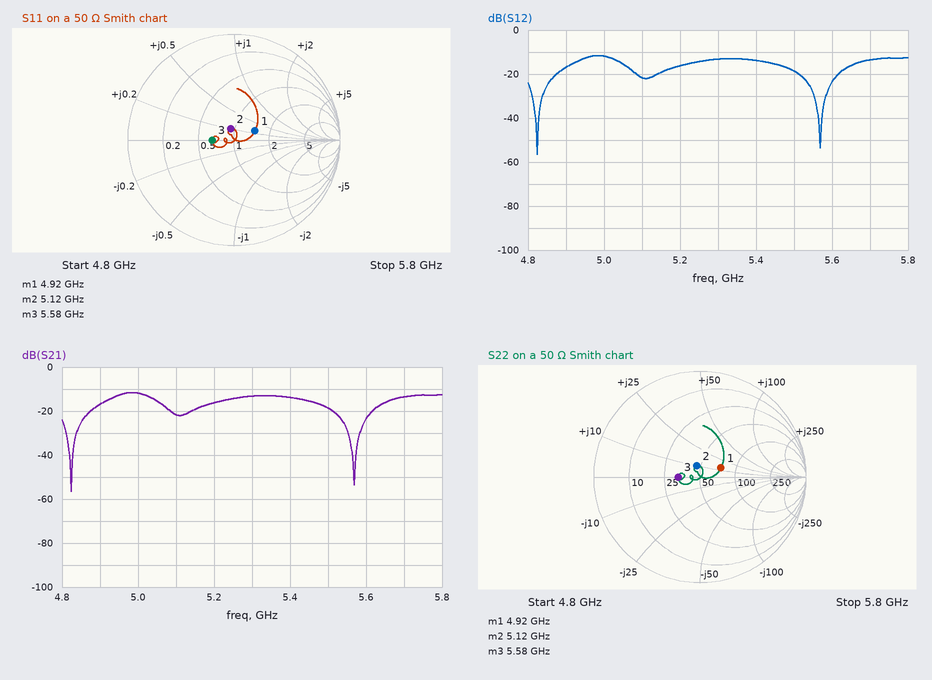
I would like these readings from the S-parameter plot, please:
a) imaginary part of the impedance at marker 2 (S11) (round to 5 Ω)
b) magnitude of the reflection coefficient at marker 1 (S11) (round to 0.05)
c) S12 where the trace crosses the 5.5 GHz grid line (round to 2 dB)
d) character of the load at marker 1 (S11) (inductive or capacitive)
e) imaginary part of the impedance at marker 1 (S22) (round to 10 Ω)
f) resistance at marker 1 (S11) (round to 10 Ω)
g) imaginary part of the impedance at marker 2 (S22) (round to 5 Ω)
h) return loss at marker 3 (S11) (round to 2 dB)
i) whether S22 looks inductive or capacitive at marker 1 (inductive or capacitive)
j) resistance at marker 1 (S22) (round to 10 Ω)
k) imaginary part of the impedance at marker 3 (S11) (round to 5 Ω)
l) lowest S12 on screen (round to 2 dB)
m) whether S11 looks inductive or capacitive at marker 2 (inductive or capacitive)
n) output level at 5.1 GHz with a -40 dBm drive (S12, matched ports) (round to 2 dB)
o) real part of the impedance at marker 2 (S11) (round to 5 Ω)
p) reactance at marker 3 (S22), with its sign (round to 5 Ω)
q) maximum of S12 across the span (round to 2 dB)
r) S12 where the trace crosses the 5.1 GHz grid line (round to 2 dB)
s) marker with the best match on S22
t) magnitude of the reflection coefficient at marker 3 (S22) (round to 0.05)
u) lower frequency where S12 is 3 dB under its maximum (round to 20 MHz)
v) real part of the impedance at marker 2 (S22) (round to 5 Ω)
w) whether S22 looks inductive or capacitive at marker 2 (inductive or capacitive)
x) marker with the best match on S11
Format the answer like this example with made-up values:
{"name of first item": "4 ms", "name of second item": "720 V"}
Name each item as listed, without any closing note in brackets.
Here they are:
{"imaginary part of the impedance at marker 2 (S11)": "+10 Ω", "magnitude of the reflection coefficient at marker 1 (S11)": "0.20", "S12 where the trace crosses the 5.5 GHz grid line": "-18 dB", "character of the load at marker 1 (S11)": "inductive", "imaginary part of the impedance at marker 1 (S22)": "+10 Ω", "resistance at marker 1 (S11)": "70 Ω", "imaginary part of the impedance at marker 2 (S22)": "+10 Ω", "return loss at marker 3 (S11)": "14 dB", "whether S22 looks inductive or capacitive at marker 1": "inductive", "resistance at marker 1 (S22)": "70 Ω", "imaginary part of the impedance at marker 3 (S11)": "0 Ω", "lowest S12 on screen": "-56 dB", "whether S11 looks inductive or capacitive at marker 2": "inductive", "output level at 5.1 GHz with a -40 dBm drive (S12, matched ports)": "-62 dBm", "real part of the impedance at marker 2 (S11)": "45 Ω", "reactance at marker 3 (S22), with its sign": "0 Ω", "maximum of S12 across the span": "-12 dB", "S12 where the trace crosses the 5.1 GHz grid line": "-22 dB", "marker with the best match on S22": "marker 2", "magnitude of the reflection coefficient at marker 3 (S22)": "0.20", "lower frequency where S12 is 3 dB under its maximum": "4.92 GHz", "real part of the impedance at marker 2 (S22)": "45 Ω", "whether S22 looks inductive or capacitive at marker 2": "inductive", "marker with the best match on S11": "marker 2"}
